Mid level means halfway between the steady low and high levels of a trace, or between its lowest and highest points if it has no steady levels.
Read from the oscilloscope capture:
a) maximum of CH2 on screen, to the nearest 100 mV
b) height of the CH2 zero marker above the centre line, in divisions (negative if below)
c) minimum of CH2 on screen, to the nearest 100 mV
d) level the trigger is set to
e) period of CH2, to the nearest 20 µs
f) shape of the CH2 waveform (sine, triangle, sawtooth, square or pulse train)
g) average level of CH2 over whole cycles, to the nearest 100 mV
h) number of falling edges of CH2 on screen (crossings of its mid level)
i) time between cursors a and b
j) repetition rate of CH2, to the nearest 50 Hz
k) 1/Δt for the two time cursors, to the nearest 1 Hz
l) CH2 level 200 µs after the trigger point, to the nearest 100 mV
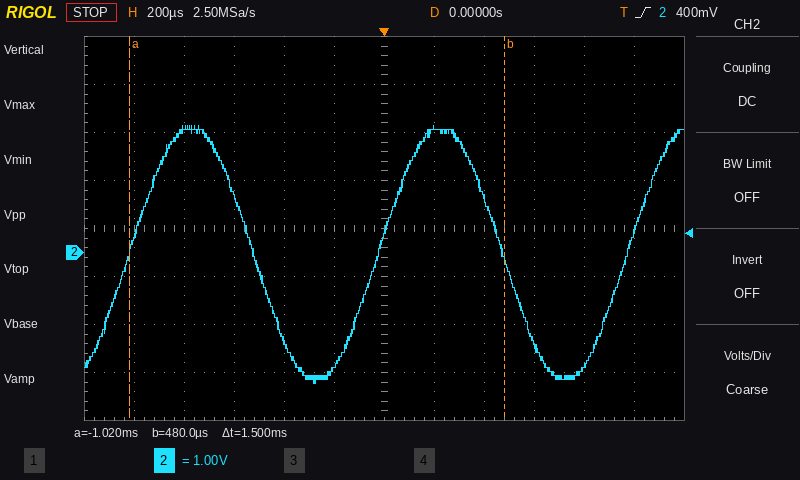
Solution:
2.6 V
-0.5 div
-2.7 V
400 mV
1.00 ms
sine
0.0 V
2
1.5 ms
1.00 kHz
667 Hz
2.6 V
